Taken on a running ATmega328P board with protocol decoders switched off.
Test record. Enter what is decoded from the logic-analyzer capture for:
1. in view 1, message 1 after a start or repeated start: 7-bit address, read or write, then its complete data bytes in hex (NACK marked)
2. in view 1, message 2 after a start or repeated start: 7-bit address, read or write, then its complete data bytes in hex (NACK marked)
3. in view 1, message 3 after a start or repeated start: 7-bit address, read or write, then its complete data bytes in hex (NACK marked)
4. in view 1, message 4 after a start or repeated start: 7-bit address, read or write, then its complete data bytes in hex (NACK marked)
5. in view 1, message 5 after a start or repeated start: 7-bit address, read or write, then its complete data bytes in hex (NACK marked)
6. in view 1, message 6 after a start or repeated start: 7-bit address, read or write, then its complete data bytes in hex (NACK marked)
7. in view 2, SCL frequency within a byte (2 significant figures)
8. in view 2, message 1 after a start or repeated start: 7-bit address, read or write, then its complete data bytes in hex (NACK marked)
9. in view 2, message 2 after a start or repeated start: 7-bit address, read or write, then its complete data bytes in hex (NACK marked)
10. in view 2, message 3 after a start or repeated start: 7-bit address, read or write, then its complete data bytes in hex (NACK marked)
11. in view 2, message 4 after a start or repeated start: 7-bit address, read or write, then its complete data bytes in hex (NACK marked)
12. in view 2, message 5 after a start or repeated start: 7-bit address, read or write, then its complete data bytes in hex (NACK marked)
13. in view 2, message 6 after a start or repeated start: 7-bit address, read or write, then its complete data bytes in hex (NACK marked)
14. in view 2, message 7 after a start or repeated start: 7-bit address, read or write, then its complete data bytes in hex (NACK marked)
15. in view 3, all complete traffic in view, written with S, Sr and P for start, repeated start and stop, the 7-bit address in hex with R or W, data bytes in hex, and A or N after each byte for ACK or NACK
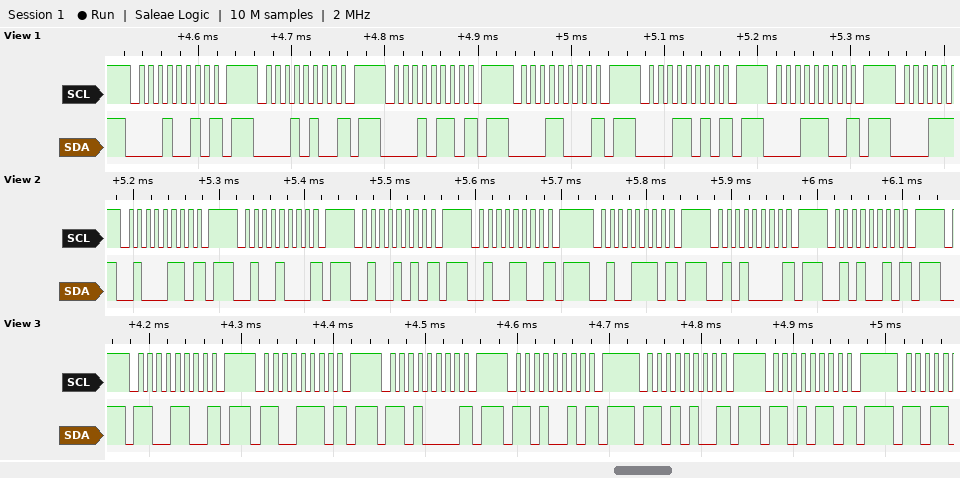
0x09 write NACK
0x0A write NACK
0x0B write NACK
0x0C write NACK
0x0D write NACK
0x0E write NACK
100 kHz
0x23 write NACK
0x24 write NACK
0x25 write NACK
0x26 write NACK
0x27 write NACK
0x28 write NACK
0x29 write NACK
S 66W N P S 67W N P S 68W N P S 69W N P S 6AW N P S 6BW N P
